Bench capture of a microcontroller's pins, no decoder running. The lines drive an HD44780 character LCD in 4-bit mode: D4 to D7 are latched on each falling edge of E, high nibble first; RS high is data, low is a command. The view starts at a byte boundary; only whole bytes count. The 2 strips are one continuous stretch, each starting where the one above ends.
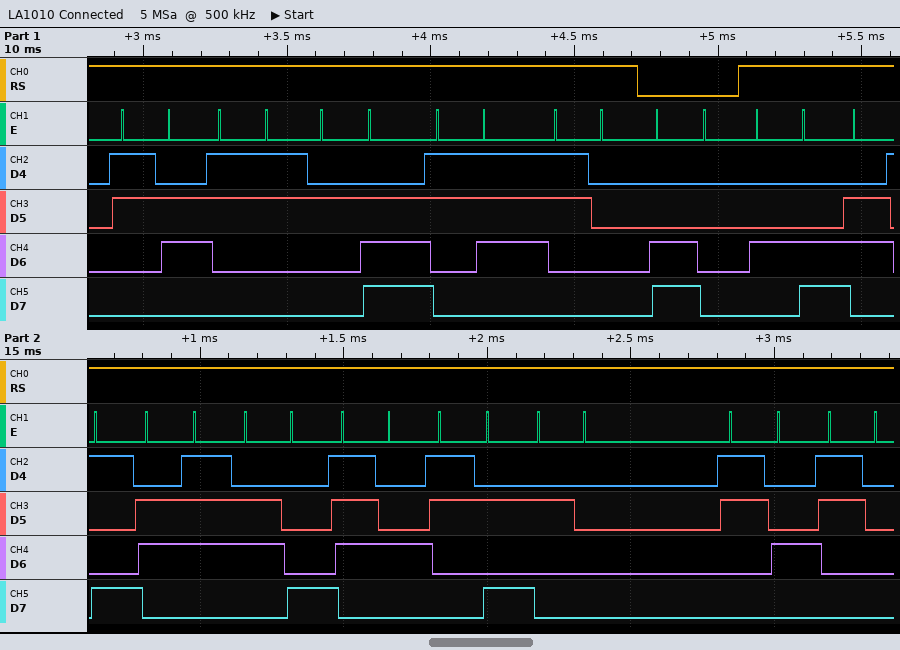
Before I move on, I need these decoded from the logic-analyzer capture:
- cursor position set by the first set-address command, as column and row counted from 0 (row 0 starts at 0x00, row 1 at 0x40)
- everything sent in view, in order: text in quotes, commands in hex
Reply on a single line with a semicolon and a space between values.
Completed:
column 0, row 1; "63.70" 0xC0 "Light: 40"
